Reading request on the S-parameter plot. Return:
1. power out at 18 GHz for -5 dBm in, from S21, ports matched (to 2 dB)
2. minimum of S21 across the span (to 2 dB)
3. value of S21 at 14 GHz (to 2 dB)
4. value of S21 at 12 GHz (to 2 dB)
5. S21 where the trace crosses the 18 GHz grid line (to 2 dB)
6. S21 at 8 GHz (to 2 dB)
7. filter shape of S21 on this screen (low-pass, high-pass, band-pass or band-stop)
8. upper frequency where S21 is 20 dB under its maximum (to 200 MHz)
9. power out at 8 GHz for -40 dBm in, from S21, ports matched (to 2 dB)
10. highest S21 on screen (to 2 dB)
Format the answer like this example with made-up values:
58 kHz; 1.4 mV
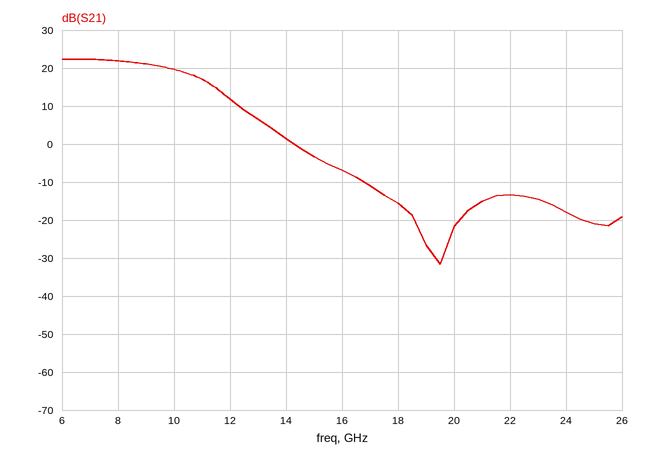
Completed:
-20 dBm; -32 dB; 2 dB; 12 dB; -16 dB; 22 dB; low-pass; 13.8 GHz; -18 dBm; 22 dB
